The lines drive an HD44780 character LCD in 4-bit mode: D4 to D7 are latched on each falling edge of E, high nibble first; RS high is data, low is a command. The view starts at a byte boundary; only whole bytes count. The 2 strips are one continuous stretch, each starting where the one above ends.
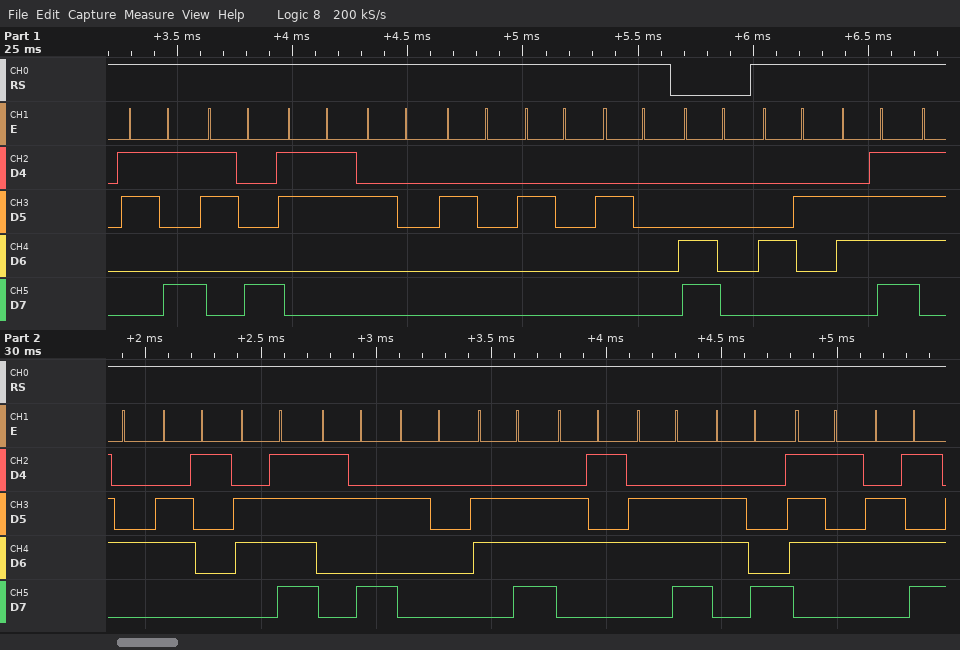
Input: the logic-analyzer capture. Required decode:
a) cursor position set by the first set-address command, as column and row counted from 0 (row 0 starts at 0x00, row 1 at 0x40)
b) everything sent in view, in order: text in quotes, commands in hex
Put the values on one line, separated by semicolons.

column 0, row 1; "983    " 0xC0 "Botao: nenhum"
